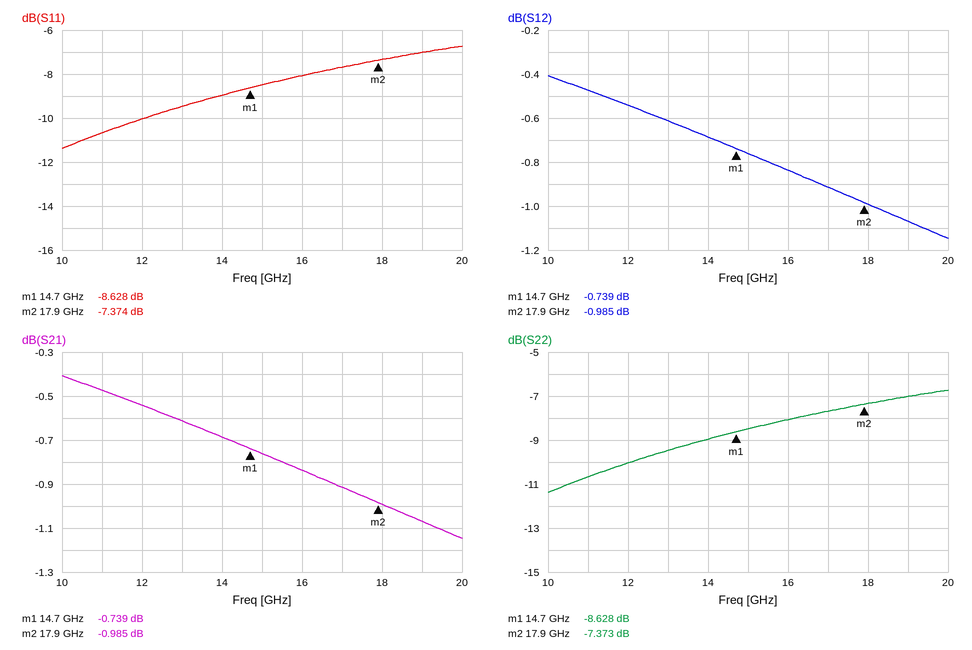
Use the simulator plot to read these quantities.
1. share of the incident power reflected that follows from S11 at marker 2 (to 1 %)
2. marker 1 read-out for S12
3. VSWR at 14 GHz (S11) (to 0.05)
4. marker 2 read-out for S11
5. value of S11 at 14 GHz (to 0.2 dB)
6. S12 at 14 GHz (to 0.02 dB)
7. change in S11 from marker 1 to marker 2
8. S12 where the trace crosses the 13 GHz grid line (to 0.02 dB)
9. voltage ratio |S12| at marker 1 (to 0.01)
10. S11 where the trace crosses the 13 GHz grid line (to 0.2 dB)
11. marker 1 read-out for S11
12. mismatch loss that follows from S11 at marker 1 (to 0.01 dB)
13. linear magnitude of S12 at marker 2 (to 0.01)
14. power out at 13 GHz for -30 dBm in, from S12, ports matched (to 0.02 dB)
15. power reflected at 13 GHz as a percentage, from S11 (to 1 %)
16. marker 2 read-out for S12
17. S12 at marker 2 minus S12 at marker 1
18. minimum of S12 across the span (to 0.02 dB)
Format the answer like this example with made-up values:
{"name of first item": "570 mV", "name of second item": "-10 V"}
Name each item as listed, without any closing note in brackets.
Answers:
{"share of the incident power reflected that follows from S11 at marker 2": "18 %", "marker 1 read-out for S12": "-0.739 dB", "VSWR at 14 GHz (S11)": "2.10", "marker 2 read-out for S11": "-7.374 dB", "value of S11 at 14 GHz": "-9.0 dB", "S12 at 14 GHz": "-0.68 dB", "change in S11 from marker 1 to marker 2": "1.254 dB", "S12 where the trace crosses the 13 GHz grid line": "-0.62 dB", "voltage ratio |S12| at marker 1": "0.92", "S11 where the trace crosses the 13 GHz grid line": "-9.4 dB", "marker 1 read-out for S11": "-8.628 dB", "mismatch loss that follows from S11 at marker 1": "0.64 dB", "linear magnitude of S12 at marker 2": "0.89", "power out at 13 GHz for -30 dBm in, from S12, ports matched": "-30.62 dBm", "power reflected at 13 GHz as a percentage, from S11": "11 %", "marker 2 read-out for S12": "-0.985 dB", "S12 at marker 2 minus S12 at marker 1": "-0.246 dB", "minimum of S12 across the span": "-1.14 dB"}
